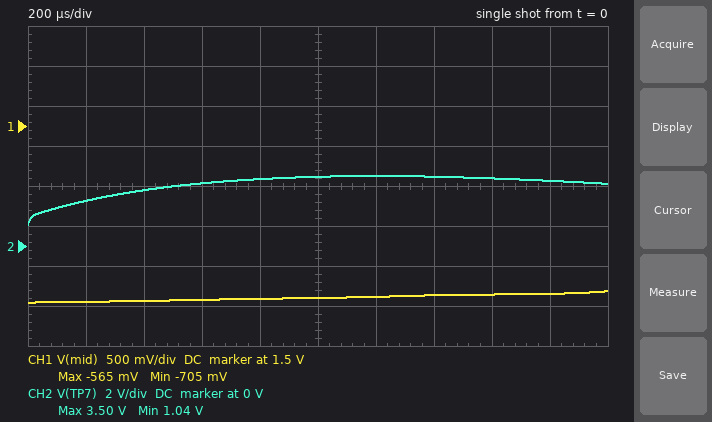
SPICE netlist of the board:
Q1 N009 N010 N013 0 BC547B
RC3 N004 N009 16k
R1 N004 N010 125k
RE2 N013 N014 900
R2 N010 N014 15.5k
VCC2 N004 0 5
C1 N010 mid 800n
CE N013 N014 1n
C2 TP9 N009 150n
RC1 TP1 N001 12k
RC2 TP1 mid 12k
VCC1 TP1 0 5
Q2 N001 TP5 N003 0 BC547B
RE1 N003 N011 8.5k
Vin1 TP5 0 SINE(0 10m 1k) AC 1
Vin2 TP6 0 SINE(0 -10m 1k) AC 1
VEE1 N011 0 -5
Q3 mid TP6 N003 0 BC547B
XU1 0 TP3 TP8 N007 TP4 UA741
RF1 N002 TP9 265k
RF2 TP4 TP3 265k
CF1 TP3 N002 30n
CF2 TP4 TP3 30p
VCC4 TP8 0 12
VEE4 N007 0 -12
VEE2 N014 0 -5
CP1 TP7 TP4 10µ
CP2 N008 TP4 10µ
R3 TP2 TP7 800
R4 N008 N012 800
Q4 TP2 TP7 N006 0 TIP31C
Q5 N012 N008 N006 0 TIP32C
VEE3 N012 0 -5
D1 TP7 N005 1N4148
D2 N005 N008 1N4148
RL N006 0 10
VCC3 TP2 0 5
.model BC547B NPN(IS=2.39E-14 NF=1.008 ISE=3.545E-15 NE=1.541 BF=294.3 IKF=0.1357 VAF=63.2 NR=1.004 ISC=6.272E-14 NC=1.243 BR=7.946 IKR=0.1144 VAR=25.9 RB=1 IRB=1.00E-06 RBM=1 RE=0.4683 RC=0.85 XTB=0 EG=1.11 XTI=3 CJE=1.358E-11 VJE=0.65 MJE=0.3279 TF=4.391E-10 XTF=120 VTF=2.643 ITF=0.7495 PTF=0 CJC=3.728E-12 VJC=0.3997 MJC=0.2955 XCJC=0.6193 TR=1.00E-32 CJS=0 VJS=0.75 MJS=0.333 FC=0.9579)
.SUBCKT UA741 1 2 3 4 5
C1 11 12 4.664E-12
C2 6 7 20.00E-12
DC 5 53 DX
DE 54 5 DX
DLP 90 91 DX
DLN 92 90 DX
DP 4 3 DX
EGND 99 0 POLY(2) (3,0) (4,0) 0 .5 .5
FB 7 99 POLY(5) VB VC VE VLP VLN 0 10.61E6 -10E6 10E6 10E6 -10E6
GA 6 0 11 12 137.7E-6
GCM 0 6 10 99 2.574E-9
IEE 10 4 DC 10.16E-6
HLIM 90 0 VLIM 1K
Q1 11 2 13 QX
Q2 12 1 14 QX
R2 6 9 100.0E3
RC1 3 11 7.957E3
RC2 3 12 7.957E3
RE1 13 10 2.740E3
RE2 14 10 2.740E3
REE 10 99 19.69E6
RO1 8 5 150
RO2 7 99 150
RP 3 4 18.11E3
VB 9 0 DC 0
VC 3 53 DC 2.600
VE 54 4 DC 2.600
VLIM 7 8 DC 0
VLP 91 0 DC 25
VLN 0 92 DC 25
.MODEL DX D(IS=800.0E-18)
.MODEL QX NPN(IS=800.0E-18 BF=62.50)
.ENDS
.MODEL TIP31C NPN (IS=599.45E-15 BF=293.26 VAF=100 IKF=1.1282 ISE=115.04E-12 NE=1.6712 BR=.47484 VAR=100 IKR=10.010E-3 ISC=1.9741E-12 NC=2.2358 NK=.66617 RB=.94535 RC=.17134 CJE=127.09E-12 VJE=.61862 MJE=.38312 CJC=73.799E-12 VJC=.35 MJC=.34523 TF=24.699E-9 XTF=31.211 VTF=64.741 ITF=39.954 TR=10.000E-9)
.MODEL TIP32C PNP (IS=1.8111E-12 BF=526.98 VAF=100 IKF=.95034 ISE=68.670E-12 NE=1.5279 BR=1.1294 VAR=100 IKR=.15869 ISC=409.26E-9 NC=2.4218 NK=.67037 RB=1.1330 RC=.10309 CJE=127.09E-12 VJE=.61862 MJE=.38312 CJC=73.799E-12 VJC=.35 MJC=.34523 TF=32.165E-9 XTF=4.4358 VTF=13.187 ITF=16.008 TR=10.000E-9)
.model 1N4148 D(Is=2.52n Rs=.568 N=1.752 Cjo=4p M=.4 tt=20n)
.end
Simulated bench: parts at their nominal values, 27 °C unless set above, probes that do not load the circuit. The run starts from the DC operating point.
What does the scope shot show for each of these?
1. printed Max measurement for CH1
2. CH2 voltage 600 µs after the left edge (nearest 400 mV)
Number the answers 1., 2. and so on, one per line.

1. -565 mV
2. 3.2 V
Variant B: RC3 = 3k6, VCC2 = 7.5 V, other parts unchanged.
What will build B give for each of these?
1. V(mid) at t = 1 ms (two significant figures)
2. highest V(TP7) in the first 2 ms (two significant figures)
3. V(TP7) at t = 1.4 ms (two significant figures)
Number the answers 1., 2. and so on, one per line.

1. -600 mV
2. 2.3 V
3. 2.2 V
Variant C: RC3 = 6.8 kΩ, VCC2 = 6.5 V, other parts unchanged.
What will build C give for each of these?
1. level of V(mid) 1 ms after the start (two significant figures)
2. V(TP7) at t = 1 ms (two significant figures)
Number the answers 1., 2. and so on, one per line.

1. -630 mV
2. 3.0 V
